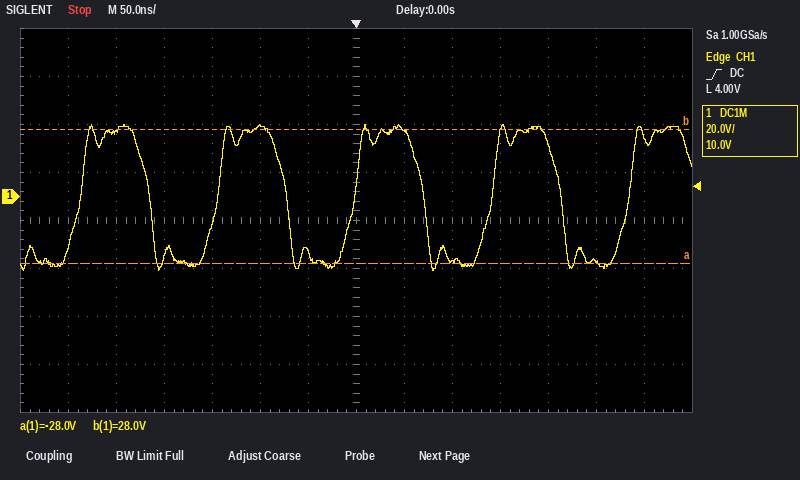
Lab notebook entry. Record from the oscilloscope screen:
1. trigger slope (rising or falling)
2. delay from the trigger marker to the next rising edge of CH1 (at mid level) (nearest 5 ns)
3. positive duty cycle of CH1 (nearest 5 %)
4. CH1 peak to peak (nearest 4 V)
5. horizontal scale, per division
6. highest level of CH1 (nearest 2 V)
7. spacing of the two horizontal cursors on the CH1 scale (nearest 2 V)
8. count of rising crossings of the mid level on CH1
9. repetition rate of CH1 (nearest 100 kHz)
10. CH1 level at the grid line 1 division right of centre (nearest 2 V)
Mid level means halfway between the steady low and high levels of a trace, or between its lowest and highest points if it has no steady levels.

rising
140 ns
50 %
60 V
50 ns
30 V
56 V
5
7.0 MHz
28 V
